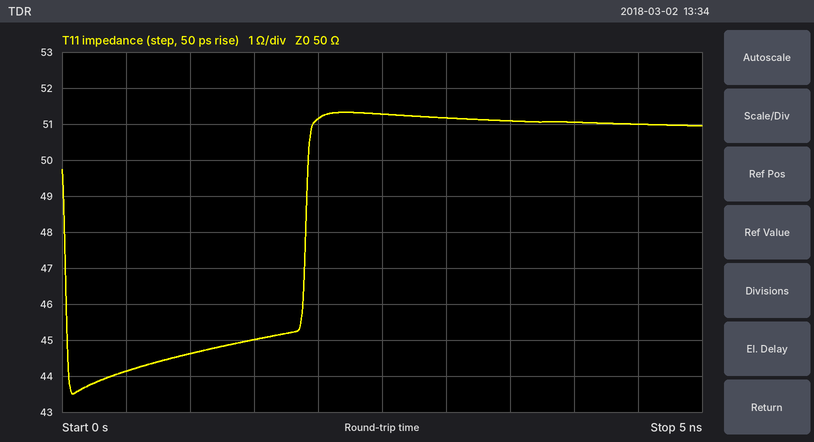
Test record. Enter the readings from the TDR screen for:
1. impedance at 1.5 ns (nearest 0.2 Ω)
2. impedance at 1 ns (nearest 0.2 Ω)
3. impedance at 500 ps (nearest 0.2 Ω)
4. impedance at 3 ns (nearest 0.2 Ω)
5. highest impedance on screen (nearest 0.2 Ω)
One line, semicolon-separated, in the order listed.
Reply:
45.0 Ω; 44.6 Ω; 44.2 Ω; 51.2 Ω; 51.4 Ω
